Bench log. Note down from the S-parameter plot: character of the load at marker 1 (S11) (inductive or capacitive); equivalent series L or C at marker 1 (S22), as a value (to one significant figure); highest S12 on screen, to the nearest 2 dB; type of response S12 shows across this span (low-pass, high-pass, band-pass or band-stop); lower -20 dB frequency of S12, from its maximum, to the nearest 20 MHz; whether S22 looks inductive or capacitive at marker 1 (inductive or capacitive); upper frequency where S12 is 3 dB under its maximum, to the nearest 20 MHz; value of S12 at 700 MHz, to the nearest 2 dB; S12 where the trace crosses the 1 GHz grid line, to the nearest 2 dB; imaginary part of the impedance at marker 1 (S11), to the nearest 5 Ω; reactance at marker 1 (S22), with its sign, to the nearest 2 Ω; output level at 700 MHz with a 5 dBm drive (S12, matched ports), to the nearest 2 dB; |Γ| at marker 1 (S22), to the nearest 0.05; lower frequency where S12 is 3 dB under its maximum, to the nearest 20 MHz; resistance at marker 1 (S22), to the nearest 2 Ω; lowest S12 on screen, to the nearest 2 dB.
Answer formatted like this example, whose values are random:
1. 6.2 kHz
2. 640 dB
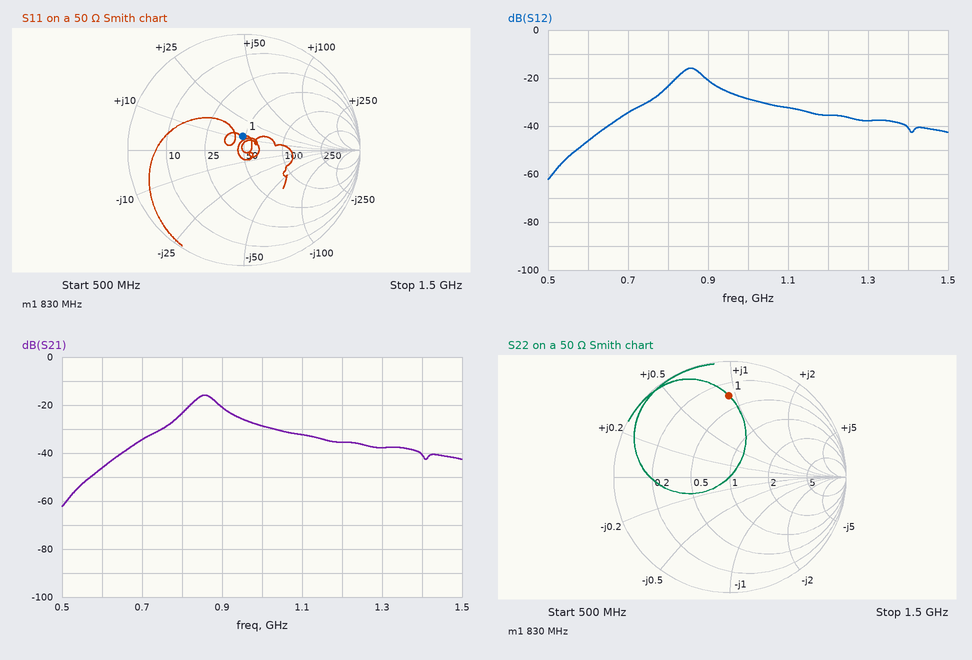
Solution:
1. inductive
2. 9 nH
3. -16 dB
4. band-pass
5. 680 MHz
6. inductive
7. 880 MHz
8. -34 dB
9. -28 dB
10. +10 Ω
11. +46 Ω
12. -30 dBm
13. 0.70
14. 820 MHz
15. 16 Ω
16. -62 dB
